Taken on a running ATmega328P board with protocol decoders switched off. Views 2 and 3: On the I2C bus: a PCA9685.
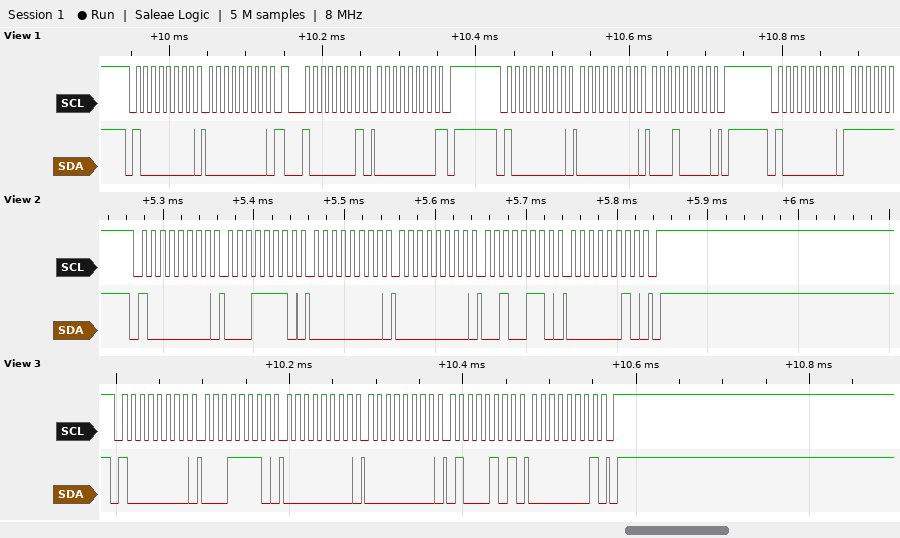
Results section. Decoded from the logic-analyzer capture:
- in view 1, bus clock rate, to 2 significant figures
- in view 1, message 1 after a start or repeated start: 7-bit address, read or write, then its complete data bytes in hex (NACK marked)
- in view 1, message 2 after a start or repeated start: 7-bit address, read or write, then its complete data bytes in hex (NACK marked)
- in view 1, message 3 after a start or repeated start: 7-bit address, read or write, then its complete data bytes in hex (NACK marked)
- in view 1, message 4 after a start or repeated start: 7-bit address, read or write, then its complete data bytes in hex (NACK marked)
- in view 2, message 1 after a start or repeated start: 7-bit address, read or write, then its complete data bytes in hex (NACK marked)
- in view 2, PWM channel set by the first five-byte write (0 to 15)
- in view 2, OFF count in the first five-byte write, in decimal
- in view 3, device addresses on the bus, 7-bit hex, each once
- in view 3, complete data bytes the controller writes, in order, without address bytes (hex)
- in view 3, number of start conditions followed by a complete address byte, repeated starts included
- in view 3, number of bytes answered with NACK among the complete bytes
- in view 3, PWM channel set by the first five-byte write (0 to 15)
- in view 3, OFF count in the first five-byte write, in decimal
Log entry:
100 kHz
0x40 write: 00
0x40 read: 00 NACK
0x40 write: 00 10
0x40 write
0x40 write: 1E 00 00 26 02
6
550
0x40
1E 00 00 45 01
1
0
6
325
